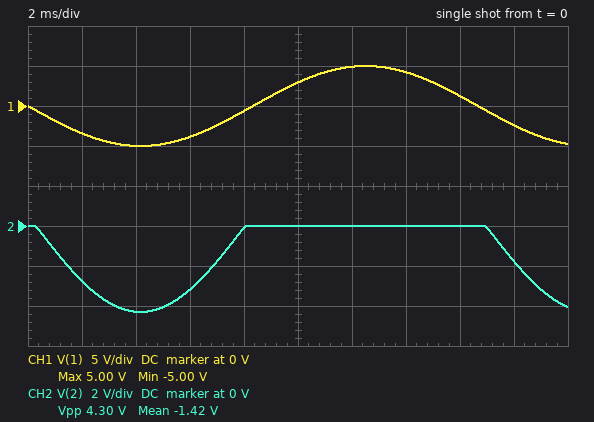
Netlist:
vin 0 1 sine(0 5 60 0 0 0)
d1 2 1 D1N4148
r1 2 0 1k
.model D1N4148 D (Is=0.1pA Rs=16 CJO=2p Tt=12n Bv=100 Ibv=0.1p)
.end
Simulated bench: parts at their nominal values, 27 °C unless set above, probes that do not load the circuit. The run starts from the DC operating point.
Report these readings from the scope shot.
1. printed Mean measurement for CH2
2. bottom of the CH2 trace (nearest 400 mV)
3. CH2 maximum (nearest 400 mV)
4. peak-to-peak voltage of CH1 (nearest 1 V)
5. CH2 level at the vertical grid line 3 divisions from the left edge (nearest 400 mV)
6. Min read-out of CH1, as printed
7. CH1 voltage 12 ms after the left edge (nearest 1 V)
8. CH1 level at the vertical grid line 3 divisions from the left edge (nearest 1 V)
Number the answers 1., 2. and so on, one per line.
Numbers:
1. -1.42 V
2. -4.4 V
3. 0 V
4. 10 V
5. -3.2 V
6. -5.00 V
7. 5 V
8. -4 V
